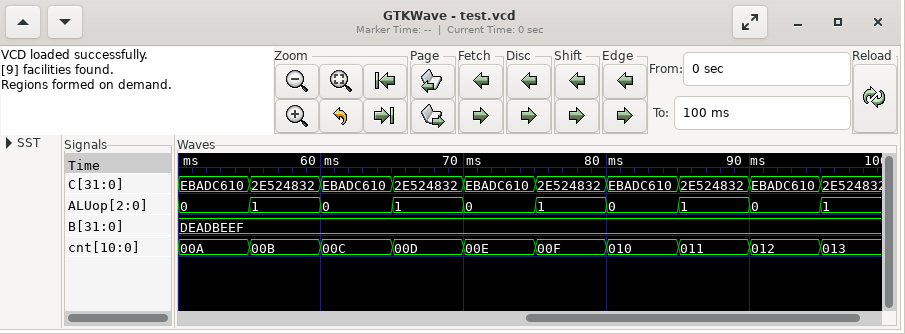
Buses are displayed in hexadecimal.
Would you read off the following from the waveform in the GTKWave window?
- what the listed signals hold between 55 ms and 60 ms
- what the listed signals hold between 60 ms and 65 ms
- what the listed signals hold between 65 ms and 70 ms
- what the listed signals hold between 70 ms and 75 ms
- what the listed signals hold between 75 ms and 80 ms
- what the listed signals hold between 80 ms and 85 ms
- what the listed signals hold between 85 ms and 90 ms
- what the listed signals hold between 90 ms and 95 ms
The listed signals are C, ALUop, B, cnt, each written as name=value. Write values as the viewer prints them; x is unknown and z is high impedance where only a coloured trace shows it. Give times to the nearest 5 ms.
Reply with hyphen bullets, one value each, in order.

- C=2E524832, ALUop=1, B=DEADBEEF, cnt=00B
- C=EBADC610, ALUop=0, B=DEADBEEF, cnt=00C
- C=2E524832, ALUop=1, B=DEADBEEF, cnt=00D
- C=EBADC610, ALUop=0, B=DEADBEEF, cnt=00E
- C=2E524832, ALUop=1, B=DEADBEEF, cnt=00F
- C=EBADC610, ALUop=0, B=DEADBEEF, cnt=010
- C=2E524832, ALUop=1, B=DEADBEEF, cnt=011
- C=EBADC610, ALUop=0, B=DEADBEEF, cnt=012
